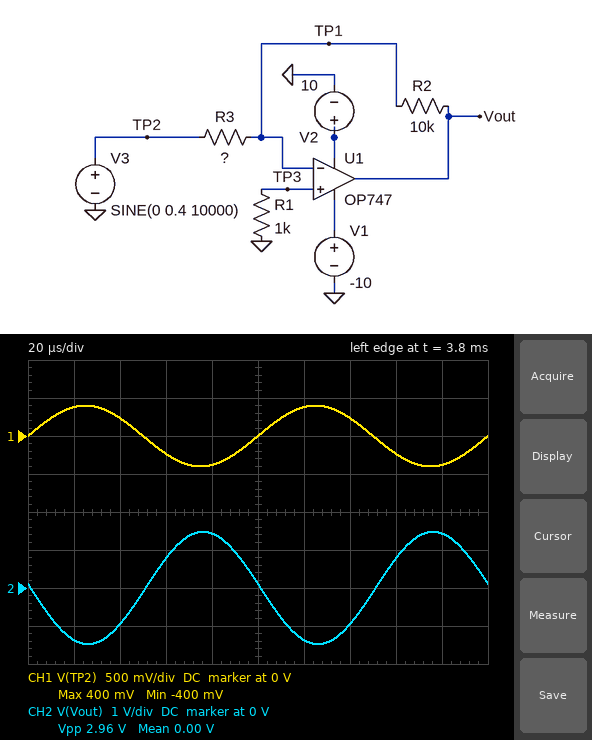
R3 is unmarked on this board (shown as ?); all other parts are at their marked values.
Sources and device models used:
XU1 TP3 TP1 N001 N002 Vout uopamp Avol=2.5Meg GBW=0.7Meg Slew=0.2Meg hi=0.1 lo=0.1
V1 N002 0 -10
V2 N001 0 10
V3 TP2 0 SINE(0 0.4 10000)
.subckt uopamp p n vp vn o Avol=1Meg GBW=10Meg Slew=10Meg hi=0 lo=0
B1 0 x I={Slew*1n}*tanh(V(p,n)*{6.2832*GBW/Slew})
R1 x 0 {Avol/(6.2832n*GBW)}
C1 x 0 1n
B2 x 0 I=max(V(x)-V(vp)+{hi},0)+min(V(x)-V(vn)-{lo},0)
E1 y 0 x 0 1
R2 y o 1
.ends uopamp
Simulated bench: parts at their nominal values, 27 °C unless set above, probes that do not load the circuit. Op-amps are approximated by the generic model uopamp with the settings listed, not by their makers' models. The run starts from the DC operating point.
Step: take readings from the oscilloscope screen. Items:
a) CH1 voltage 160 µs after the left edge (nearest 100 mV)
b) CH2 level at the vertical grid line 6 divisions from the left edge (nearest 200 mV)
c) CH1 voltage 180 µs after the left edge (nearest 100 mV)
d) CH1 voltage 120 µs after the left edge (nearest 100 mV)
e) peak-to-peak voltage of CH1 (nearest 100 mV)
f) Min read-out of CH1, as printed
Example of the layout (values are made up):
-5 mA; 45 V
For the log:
-200 mV; -1.4 V; -400 mV; 400 mV; 800 mV; -400 mV
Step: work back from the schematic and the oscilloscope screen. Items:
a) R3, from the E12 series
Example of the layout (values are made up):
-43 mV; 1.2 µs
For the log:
2.7 kΩ
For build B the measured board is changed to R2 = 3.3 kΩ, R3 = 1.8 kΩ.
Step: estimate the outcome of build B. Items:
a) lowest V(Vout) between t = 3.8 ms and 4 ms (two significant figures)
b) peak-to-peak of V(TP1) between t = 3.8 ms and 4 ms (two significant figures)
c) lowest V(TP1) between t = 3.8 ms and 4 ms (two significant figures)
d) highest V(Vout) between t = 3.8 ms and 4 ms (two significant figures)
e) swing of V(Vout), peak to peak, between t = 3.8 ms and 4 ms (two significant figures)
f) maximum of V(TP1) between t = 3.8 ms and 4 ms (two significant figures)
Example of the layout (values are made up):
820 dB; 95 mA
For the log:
-730 mV; 21 mV; -11 mV; 730 mV; 1.5 V; 11 mV
